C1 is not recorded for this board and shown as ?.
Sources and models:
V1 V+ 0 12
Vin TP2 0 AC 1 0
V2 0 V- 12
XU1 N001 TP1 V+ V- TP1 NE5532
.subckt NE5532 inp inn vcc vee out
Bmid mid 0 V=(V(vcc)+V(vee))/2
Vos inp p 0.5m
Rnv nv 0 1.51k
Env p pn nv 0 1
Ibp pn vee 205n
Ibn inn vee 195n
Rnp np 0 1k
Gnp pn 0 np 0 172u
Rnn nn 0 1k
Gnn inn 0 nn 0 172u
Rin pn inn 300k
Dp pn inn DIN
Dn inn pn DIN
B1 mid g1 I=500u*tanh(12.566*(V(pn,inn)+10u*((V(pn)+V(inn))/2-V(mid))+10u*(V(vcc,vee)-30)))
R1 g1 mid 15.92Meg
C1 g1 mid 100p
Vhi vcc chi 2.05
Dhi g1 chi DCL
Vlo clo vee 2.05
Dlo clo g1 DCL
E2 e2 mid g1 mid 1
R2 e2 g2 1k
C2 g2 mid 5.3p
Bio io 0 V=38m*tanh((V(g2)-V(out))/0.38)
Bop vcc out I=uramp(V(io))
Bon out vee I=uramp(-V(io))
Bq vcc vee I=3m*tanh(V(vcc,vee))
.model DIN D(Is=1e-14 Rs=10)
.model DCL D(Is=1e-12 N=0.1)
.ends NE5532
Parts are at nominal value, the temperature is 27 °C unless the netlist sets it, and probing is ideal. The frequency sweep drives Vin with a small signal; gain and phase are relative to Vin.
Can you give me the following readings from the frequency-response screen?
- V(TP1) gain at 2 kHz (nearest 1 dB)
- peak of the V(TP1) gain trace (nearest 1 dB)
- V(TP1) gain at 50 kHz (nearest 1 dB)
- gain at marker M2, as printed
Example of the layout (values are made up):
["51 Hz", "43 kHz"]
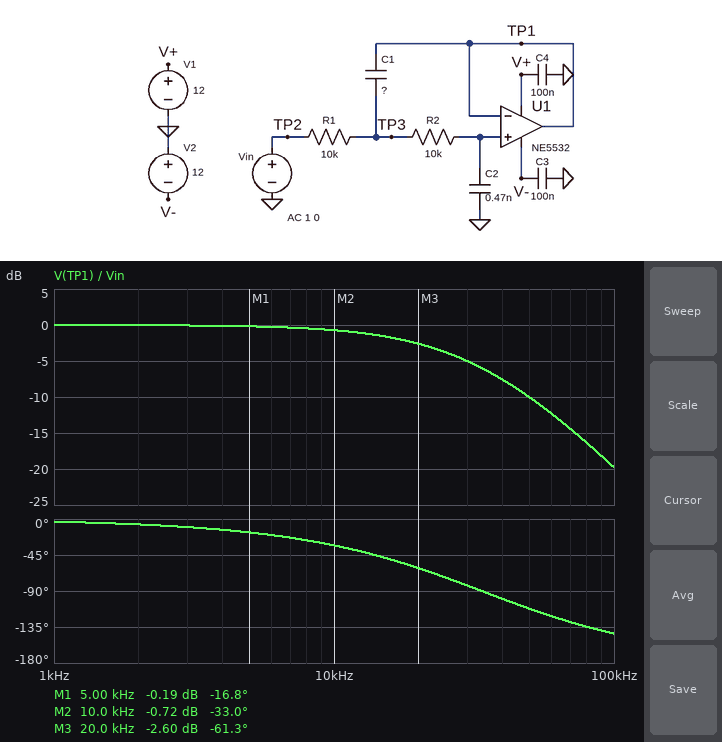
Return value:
["0 dB", "0 dB", "-10 dB", "-0.72 dB"]
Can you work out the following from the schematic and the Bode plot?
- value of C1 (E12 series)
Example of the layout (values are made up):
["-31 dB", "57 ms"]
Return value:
["470 pF"]
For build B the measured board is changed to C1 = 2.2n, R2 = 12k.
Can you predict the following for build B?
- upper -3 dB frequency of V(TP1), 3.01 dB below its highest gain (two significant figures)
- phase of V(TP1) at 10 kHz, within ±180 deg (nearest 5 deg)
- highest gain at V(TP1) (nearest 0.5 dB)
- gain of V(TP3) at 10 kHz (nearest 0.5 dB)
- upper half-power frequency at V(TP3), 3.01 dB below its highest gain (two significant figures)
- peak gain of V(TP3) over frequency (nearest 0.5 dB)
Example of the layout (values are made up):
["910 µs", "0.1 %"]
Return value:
["17 kHz", "-50 deg", "1.5 dB", "2.0 dB", "18 kHz", "2.5 dB"]
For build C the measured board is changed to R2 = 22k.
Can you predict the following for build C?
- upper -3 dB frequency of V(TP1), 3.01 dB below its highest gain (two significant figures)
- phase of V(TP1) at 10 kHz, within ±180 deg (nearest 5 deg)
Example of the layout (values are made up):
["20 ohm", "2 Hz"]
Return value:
["13 kHz", "-50 deg"]
